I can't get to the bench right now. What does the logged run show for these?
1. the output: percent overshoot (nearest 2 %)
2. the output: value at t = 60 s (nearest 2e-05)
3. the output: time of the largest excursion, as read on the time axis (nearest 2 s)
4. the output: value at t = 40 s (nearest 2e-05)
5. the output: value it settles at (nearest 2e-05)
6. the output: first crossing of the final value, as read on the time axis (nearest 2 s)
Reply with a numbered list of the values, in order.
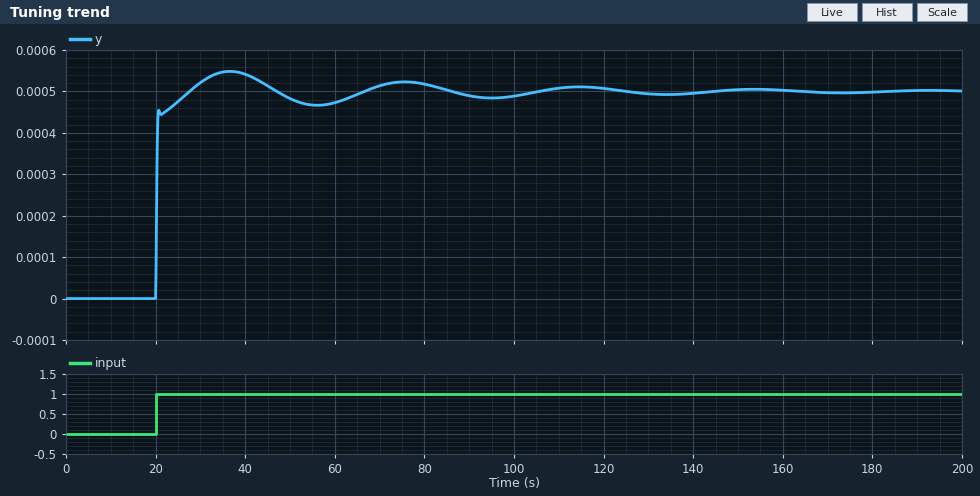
1. 10 %
2. 0.00048
3. 36 s
4. 0.00054
5. 0.00050
6. 28 s
